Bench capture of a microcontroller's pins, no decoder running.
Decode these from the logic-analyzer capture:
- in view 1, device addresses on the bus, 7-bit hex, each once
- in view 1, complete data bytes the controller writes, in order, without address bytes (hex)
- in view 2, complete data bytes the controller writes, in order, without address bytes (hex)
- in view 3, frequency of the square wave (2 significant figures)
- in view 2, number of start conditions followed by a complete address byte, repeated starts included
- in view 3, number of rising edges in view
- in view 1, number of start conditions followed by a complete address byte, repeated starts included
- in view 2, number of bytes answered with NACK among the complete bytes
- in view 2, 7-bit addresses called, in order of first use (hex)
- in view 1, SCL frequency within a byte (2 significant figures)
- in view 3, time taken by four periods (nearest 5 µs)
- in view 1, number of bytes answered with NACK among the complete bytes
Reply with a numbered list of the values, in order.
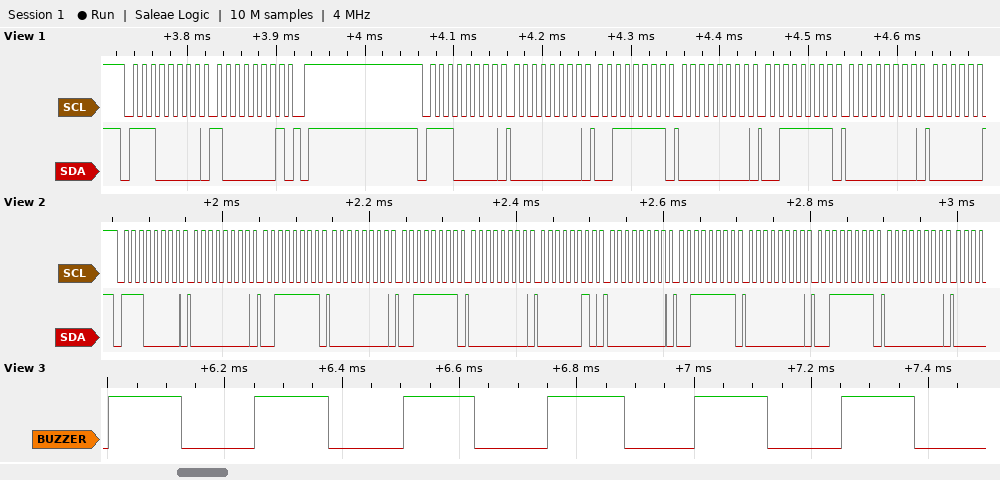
1. 0x70
2. 81 00 3F 00 3F 00
3. 00 3F 00 3F 00 02 00 3F 00 3F 00
4. 4.0 kHz
5. 1
6. 6
7. 2
8. 0
9. 0x70
10. 100 kHz
11. 1000 µs
12. 0
